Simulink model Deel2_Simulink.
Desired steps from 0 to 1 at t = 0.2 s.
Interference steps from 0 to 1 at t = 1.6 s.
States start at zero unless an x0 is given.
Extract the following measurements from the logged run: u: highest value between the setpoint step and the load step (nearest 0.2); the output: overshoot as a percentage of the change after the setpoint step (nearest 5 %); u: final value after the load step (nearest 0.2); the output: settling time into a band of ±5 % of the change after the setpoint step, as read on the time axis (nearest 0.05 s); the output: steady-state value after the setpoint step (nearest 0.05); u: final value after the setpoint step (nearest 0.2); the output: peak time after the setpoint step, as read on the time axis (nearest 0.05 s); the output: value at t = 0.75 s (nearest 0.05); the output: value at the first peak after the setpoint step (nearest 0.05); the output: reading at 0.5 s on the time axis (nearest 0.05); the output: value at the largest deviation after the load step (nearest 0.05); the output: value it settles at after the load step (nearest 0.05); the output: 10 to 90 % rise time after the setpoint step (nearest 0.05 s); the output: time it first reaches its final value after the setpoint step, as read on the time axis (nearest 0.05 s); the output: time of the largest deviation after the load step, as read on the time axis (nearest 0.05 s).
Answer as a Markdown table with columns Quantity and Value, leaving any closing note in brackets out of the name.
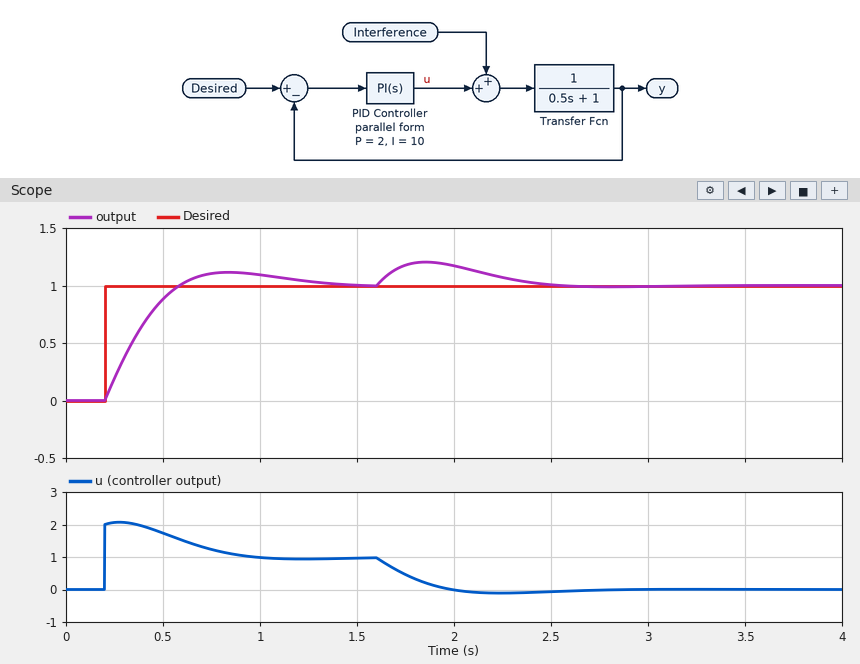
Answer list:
| Quantity | Value |
|---|---|
| u: highest value between the setpoint step and the load step | 2.0 |
| the output: overshoot as a percentage of the change after the setpoint step | 10 % |
| u: final value after the load step | 0.0 |
| the output: settling time into a band of ±5 % of the change after the setpoint step, as read on the time axis | 1.20 s |
| the output: steady-state value after the setpoint step | 1.00 |
| u: final value after the setpoint step | 1.0 |
| the output: peak time after the setpoint step, as read on the time axis | 0.85 s |
| the output: value at t = 0.75 s | 1.10 |
| the output: value at the first peak after the setpoint step | 1.10 |
| the output: reading at 0.5 s on the time axis | 0.90 |
| the output: value at the largest deviation after the load step | 1.20 |
| the output: value it settles at after the load step | 1.00 |
| the output: 10 to 90 % rise time after the setpoint step | 0.30 s |
| the output: time it first reaches its final value after the setpoint step, as read on the time axis | 0.60 s |
| the output: time of the largest deviation after the load step, as read on the time axis | 1.85 s |
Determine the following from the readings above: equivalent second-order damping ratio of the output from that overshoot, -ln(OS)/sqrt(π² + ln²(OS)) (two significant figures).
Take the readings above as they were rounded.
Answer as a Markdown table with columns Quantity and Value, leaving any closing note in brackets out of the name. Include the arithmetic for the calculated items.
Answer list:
| Quantity | Value |
|---|---|
| equivalent second-order damping ratio of the output from that overshoot, -ln(OS)/sqrt(π² + ln²(OS)) | ln(0.1) = -2.303; 2.303 / sqrt(9.870 + 5.302) = 0.59 |
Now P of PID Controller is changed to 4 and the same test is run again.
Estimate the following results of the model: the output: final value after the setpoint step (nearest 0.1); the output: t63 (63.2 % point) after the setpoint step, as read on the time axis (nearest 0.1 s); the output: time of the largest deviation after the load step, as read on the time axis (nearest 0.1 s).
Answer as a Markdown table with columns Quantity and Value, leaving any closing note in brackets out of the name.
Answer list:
| Quantity | Value |
|---|---|
| the output: final value after the setpoint step | 1.0 |
| the output: t63 (63.2 % point) after the setpoint step, as read on the time axis | 0.3 s |
| the output: time of the largest deviation after the load step, as read on the time axis | 1.8 s |
